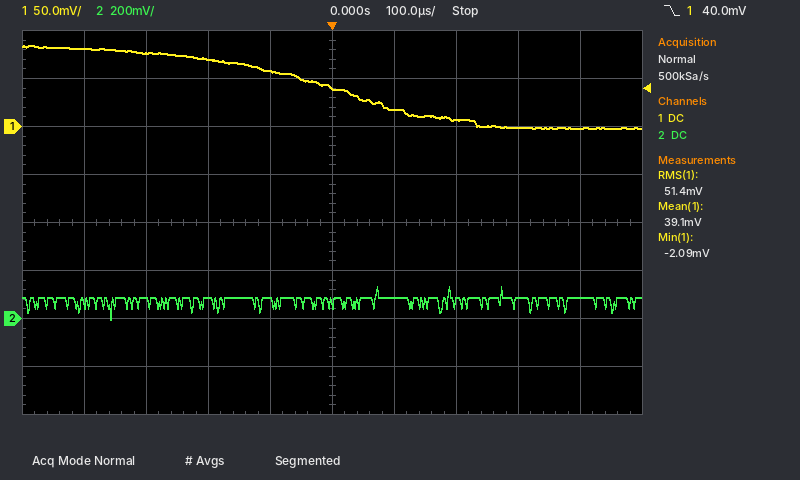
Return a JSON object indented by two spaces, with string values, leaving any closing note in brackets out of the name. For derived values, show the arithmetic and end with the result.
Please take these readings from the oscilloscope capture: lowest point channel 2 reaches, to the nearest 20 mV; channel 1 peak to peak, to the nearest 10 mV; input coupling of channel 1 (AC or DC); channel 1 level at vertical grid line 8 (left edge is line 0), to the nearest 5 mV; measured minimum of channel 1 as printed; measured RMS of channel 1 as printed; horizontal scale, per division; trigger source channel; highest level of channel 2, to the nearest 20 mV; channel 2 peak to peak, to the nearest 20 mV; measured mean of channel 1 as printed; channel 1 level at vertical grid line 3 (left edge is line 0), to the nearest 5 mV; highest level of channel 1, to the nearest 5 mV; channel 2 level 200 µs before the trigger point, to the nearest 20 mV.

{
  "lowest point channel 2 reaches, to the nearest 20 mV": "0 mV",
  "channel 1 peak to peak, to the nearest 10 mV": "90 mV",
  "input coupling of channel 1": "DC",
  "channel 1 level at vertical grid line 8 (left edge is line 0), to the nearest 5 mV": "0 mV",
  "measured minimum of channel 1 as printed": "-2.09 mV",
  "measured RMS of channel 1 as printed": "51.4 mV",
  "horizontal scale, per division": "100 µs",
  "trigger source channel": "channel 1",
  "highest level of channel 2, to the nearest 20 mV": "140 mV",
  "channel 2 peak to peak, to the nearest 20 mV": "140 mV − (0 mV) = 140 mV",
  "measured mean of channel 1 as printed": "39.1 mV",
  "channel 1 level at vertical grid line 3 (left edge is line 0), to the nearest 5 mV": "70 mV",
  "highest level of channel 1, to the nearest 5 mV": "85 mV",
  "channel 2 level 200 µs before the trigger point, to the nearest 20 mV": "80 mV"
}
